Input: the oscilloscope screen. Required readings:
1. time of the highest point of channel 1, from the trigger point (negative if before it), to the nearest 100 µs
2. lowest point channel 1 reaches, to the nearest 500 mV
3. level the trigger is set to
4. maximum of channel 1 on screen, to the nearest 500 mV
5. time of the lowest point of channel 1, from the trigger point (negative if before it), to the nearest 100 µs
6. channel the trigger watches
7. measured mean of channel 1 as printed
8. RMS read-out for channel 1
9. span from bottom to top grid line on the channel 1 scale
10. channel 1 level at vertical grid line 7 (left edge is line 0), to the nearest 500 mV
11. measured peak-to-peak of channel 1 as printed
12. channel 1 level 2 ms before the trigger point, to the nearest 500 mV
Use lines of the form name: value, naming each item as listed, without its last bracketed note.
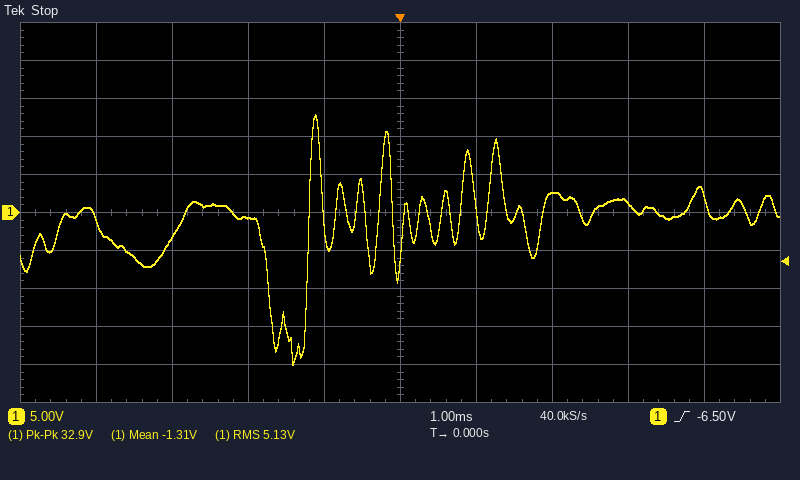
time of the highest point of channel 1, from the trigger point (negative if before it), to the nearest 100 µs: -1.1 ms
lowest point channel 1 reaches, to the nearest 500 mV: -20.0 V
level the trigger is set to: -6.50 V
maximum of channel 1 on screen, to the nearest 500 mV: 13.0 V
time of the lowest point of channel 1, from the trigger point (negative if before it), to the nearest 100 µs: -1.4 ms
channel the trigger watches: channel 1
measured mean of channel 1 as printed: -1.31 V
RMS read-out for channel 1: 5.13 V
span from bottom to top grid line on the channel 1 scale: 50 V
channel 1 level at vertical grid line 7 (left edge is line 0), to the nearest 500 mV: 2.5 V
measured peak-to-peak of channel 1 as printed: 32.9 V
channel 1 level 2 ms before the trigger point, to the nearest 500 mV: -500 mV
